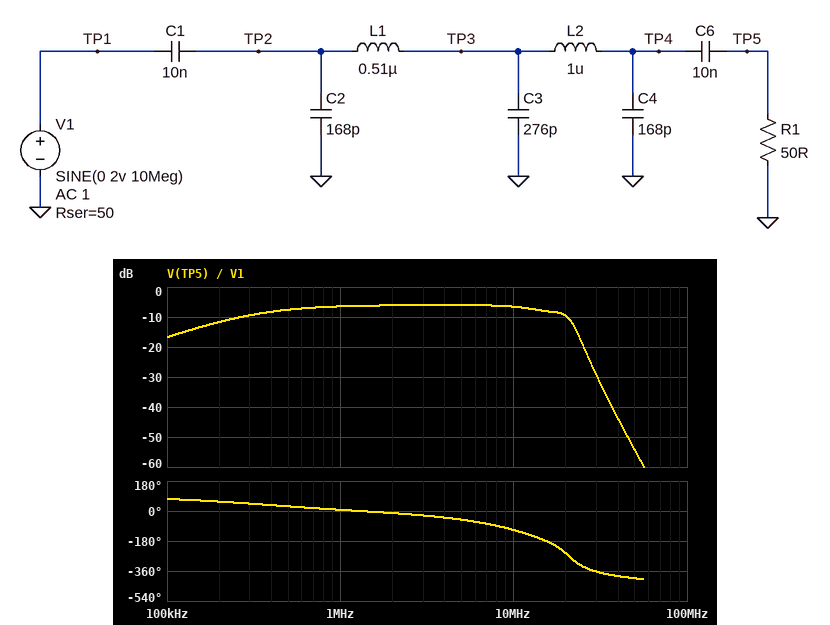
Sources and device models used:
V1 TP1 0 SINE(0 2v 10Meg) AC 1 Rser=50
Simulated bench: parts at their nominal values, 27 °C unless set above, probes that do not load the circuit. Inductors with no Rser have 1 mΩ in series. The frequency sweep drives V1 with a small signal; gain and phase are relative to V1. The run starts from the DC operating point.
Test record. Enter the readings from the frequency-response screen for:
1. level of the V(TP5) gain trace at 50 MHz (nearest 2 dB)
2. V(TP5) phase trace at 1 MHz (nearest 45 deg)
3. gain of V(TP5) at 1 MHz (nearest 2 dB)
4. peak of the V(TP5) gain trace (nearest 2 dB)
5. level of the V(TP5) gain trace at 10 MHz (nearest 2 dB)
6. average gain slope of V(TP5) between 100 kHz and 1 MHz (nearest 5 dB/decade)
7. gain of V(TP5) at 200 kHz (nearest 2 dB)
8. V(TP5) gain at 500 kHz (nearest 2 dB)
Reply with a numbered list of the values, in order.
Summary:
1. -54 dB
2. 0 deg
3. -6 dB
4. -6 dB
5. -6 dB
6. 10 dB/decade
7. -12 dB
8. -8 dB
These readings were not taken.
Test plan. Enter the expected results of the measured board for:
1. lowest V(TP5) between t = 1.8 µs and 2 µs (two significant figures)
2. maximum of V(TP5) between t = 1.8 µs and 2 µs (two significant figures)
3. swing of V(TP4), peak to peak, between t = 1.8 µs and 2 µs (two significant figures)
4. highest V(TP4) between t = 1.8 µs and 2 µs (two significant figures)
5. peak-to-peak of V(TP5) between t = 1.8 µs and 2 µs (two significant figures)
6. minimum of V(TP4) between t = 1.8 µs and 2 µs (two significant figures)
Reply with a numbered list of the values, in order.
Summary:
1. -940 mV
2. 940 mV
3. 1.9 V
4. 940 mV
5. 1.9 V
6. -940 mV
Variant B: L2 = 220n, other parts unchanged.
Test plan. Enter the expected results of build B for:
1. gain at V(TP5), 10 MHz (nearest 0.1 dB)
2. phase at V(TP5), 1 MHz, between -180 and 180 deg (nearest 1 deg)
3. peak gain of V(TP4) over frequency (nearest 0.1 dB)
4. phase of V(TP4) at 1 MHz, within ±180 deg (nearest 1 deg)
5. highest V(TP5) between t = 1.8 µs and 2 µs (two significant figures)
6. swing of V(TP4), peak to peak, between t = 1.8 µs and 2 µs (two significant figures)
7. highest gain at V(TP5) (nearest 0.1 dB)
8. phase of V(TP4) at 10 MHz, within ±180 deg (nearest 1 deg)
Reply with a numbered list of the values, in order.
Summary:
1. -6.4 dB
2. 10 deg
3. -6.2 dB
4. -8 deg
5. 950 mV
6. 1.9 V
7. -6.3 dB
8. -79 deg
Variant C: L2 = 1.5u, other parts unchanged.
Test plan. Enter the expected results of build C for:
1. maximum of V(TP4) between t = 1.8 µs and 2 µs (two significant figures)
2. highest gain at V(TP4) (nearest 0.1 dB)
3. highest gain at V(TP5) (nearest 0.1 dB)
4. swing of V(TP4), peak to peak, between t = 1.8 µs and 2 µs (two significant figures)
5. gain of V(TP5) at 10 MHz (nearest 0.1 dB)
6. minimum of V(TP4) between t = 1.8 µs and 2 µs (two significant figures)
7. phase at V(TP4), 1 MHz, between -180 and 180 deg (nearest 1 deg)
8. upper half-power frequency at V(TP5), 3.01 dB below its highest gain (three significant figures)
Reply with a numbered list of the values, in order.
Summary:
1. 780 mV
2. -5.9 dB
3. -6.0 dB
4. 1.6 V
5. -8.2 dB
6. -780 mV
7. -12 deg
8. 11.5 MHz
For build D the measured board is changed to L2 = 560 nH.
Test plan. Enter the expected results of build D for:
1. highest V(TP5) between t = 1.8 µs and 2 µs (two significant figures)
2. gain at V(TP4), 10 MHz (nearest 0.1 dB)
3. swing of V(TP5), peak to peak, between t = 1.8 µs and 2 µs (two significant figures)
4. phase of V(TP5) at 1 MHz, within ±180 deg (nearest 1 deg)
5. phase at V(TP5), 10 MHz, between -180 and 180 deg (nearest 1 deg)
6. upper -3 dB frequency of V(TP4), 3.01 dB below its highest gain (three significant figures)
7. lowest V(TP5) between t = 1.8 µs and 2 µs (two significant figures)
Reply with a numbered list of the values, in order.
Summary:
1. 1.0 V
2. -6.0 dB
3. 2.0 V
4. 9 deg
5. -93 deg
6. 24.2 MHz
7. -1.0 V
